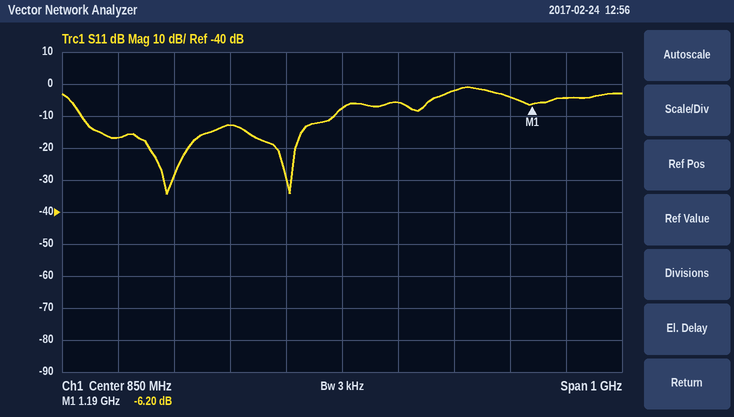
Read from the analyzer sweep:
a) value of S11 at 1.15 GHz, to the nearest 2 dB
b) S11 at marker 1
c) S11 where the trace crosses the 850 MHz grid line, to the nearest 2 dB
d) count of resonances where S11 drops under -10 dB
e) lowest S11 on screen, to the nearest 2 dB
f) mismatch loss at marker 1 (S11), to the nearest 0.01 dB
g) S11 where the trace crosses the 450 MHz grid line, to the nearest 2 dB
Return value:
-4 dB
-6.20 dB
-8 dB
2
-34 dB
1.19 dB
-16 dB
